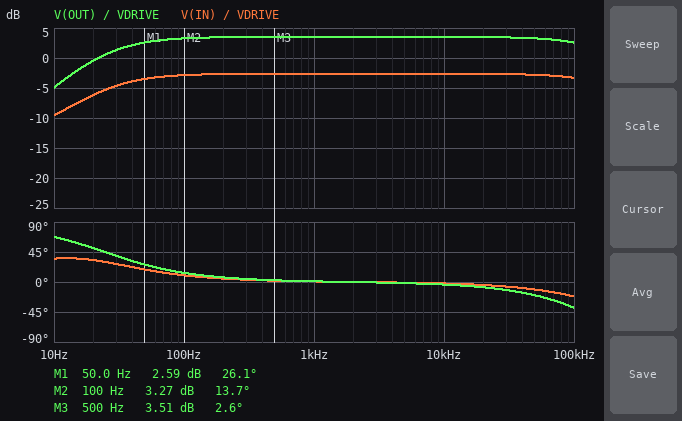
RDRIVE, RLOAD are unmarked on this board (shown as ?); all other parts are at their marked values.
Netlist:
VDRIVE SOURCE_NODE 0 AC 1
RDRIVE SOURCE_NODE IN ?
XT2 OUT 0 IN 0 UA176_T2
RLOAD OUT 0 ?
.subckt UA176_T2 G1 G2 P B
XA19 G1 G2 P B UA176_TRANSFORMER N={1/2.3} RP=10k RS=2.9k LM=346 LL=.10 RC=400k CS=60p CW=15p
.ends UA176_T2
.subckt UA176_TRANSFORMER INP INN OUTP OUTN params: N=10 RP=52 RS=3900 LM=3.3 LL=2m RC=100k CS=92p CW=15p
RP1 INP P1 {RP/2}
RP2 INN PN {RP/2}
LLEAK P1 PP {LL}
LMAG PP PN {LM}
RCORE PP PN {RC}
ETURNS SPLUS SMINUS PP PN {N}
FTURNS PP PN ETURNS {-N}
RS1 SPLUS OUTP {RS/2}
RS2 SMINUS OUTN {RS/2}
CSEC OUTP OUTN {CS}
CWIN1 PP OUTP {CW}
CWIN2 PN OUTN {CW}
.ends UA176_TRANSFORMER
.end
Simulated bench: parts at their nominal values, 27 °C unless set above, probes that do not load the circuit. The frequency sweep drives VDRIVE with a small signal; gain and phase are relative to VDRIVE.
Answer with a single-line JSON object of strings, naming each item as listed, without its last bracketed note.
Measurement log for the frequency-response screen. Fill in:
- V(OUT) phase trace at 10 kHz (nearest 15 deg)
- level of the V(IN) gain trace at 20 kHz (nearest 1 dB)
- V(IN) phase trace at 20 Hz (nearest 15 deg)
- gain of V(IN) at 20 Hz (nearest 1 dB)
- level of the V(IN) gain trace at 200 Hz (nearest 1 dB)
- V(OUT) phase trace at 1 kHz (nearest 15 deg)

{"V(OUT) phase trace at 10 kHz": "0 deg", "level of the V(IN) gain trace at 20 kHz": "-3 dB", "V(IN) phase trace at 20 Hz": "30 deg", "gain of V(IN) at 20 Hz": "-6 dB", "level of the V(IN) gain trace at 200 Hz": "-3 dB", "V(OUT) phase trace at 1 kHz": "0 deg"}
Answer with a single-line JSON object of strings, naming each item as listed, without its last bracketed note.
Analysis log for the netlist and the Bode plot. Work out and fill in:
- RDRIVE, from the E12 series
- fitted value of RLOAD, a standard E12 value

{"RDRIVE, from the E12 series": "12 kΩ", "fitted value of RLOAD, a standard E12 value": "270 kΩ"}
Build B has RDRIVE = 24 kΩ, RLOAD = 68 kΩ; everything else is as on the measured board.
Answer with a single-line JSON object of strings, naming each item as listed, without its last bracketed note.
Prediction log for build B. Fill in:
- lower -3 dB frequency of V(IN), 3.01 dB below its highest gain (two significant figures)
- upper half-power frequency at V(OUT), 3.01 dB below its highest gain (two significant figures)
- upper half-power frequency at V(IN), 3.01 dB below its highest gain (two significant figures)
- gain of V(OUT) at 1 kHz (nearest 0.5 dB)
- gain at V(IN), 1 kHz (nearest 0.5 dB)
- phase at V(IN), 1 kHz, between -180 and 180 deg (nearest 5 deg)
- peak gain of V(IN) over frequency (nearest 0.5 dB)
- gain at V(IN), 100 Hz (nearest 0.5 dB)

{"lower -3 dB frequency of V(IN), 3.01 dB below its highest gain": "33 Hz", "upper half-power frequency at V(OUT), 3.01 dB below its highest gain": "180 kHz", "upper half-power frequency at V(IN), 3.01 dB below its highest gain": "260 kHz", "gain of V(OUT) at 1 kHz": "-4.0 dB", "gain at V(IN), 1 kHz": "-8.0 dB", "phase at V(IN), 1 kHz, between -180 and 180 deg": "0 deg", "peak gain of V(IN) over frequency": "-6.5 dB", "gain at V(IN), 100 Hz": "-8.5 dB"}
